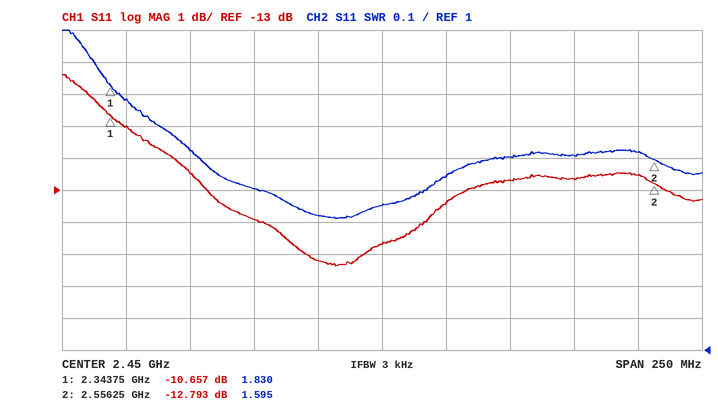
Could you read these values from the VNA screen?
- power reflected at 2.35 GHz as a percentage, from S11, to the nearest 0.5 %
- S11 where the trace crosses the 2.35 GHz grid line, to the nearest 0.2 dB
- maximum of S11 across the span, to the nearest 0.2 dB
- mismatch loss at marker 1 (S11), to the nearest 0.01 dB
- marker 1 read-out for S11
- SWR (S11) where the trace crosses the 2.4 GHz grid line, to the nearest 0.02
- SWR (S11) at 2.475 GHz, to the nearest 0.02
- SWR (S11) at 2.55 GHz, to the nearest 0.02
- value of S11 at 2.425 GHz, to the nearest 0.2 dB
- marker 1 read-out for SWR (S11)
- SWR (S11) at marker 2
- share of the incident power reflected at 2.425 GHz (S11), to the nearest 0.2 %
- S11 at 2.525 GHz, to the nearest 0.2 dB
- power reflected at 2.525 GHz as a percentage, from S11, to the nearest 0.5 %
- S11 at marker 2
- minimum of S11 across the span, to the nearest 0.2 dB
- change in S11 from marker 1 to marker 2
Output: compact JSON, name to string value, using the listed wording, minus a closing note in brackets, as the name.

{"power reflected at 2.35 GHz as a percentage, from S11, to the nearest 0.5 %": "8.0 %", "S11 where the trace crosses the 2.35 GHz grid line, to the nearest 0.2 dB": "-11.0 dB", "maximum of S11 across the span, to the nearest 0.2 dB": "-9.4 dB", "mismatch loss at marker 1 (S11), to the nearest 0.01 dB": "0.39 dB", "marker 1 read-out for S11": "-10.657 dB", "SWR (S11) where the trace crosses the 2.4 GHz grid line, to the nearest 0.02": "1.50", "SWR (S11) at 2.475 GHz, to the nearest 0.02": "1.54", "SWR (S11) at 2.55 GHz, to the nearest 0.02": "1.62", "value of S11 at 2.425 GHz, to the nearest 0.2 dB": "-15.2 dB", "marker 1 read-out for SWR": "1.830", "SWR (S11) at marker 2": "1.595", "share of the incident power reflected at 2.425 GHz (S11), to the nearest 0.2 %": "3.0 %", "S11 at 2.525 GHz, to the nearest 0.2 dB": "-12.6 dB", "power reflected at 2.525 GHz as a percentage, from S11, to the nearest 0.5 %": "5.5 %", "S11 at marker 2": "-12.793 dB", "minimum of S11 across the span, to the nearest 0.2 dB": "-15.4 dB", "change in S11 from marker 1 to marker 2": "-2.136 dB"}
